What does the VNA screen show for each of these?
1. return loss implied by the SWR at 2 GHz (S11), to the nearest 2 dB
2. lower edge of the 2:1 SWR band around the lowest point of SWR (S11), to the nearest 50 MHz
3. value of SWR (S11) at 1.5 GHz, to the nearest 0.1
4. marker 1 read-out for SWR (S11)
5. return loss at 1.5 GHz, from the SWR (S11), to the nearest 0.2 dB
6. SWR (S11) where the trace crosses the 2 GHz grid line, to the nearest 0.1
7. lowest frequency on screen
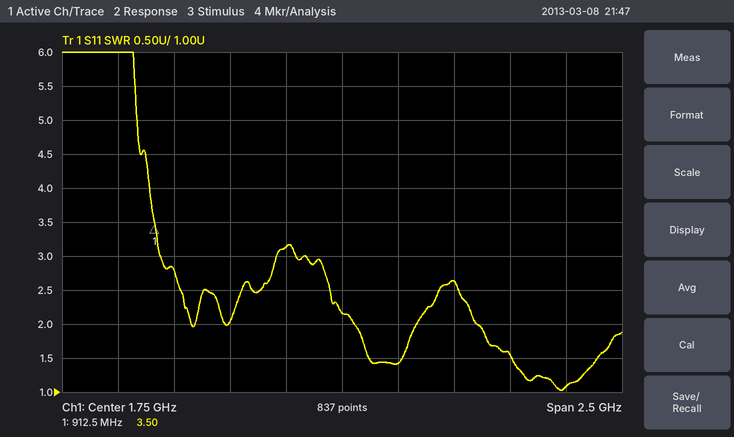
16 dB
2.35 GHz
3.1
3.50
5.8 dB
1.4
500 MHz
